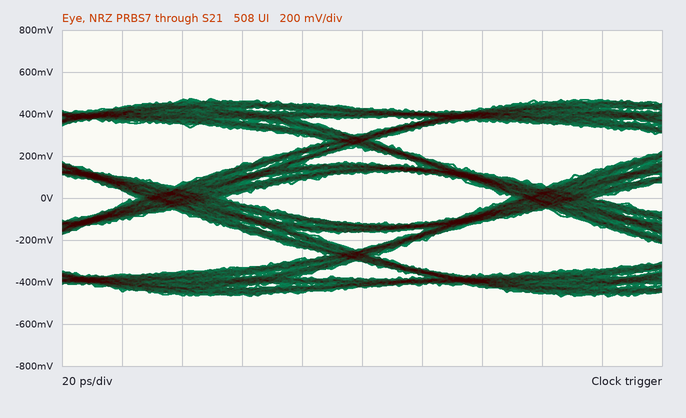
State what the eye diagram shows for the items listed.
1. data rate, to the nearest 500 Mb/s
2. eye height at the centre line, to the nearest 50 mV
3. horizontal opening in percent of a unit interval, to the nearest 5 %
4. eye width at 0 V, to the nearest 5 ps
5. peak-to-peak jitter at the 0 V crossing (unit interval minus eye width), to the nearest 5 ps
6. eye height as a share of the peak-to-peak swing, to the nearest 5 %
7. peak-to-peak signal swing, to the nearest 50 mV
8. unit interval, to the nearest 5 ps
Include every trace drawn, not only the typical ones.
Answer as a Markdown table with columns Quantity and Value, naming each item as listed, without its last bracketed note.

| Quantity | Value |
|---|---|
| data rate, to the nearest 500 Mb/s | 8.0 Gb/s |
| eye height at the centre line, to the nearest 50 mV | 250 mV |
| horizontal opening in percent of a unit interval, to the nearest 5 % | 75 % |
| eye width at 0 V, to the nearest 5 ps | 95 ps |
| peak-to-peak jitter at the 0 V crossing (unit interval minus eye width), to the nearest 5 ps | 30 ps |
| eye height as a share of the peak-to-peak swing, to the nearest 5 % | 25 % |
| peak-to-peak signal swing, to the nearest 50 mV | 950 mV |
| unit interval, to the nearest 5 ps | 125 ps |
